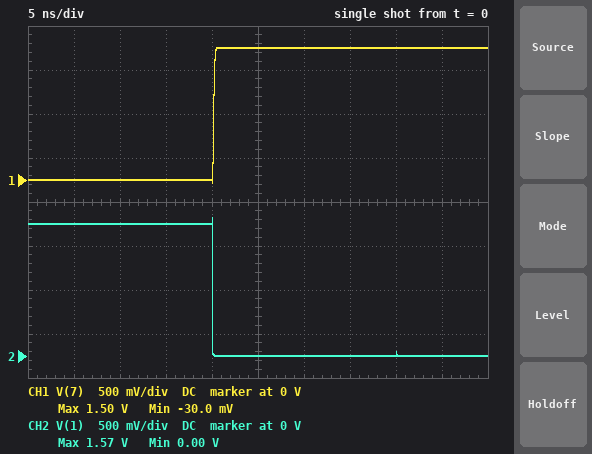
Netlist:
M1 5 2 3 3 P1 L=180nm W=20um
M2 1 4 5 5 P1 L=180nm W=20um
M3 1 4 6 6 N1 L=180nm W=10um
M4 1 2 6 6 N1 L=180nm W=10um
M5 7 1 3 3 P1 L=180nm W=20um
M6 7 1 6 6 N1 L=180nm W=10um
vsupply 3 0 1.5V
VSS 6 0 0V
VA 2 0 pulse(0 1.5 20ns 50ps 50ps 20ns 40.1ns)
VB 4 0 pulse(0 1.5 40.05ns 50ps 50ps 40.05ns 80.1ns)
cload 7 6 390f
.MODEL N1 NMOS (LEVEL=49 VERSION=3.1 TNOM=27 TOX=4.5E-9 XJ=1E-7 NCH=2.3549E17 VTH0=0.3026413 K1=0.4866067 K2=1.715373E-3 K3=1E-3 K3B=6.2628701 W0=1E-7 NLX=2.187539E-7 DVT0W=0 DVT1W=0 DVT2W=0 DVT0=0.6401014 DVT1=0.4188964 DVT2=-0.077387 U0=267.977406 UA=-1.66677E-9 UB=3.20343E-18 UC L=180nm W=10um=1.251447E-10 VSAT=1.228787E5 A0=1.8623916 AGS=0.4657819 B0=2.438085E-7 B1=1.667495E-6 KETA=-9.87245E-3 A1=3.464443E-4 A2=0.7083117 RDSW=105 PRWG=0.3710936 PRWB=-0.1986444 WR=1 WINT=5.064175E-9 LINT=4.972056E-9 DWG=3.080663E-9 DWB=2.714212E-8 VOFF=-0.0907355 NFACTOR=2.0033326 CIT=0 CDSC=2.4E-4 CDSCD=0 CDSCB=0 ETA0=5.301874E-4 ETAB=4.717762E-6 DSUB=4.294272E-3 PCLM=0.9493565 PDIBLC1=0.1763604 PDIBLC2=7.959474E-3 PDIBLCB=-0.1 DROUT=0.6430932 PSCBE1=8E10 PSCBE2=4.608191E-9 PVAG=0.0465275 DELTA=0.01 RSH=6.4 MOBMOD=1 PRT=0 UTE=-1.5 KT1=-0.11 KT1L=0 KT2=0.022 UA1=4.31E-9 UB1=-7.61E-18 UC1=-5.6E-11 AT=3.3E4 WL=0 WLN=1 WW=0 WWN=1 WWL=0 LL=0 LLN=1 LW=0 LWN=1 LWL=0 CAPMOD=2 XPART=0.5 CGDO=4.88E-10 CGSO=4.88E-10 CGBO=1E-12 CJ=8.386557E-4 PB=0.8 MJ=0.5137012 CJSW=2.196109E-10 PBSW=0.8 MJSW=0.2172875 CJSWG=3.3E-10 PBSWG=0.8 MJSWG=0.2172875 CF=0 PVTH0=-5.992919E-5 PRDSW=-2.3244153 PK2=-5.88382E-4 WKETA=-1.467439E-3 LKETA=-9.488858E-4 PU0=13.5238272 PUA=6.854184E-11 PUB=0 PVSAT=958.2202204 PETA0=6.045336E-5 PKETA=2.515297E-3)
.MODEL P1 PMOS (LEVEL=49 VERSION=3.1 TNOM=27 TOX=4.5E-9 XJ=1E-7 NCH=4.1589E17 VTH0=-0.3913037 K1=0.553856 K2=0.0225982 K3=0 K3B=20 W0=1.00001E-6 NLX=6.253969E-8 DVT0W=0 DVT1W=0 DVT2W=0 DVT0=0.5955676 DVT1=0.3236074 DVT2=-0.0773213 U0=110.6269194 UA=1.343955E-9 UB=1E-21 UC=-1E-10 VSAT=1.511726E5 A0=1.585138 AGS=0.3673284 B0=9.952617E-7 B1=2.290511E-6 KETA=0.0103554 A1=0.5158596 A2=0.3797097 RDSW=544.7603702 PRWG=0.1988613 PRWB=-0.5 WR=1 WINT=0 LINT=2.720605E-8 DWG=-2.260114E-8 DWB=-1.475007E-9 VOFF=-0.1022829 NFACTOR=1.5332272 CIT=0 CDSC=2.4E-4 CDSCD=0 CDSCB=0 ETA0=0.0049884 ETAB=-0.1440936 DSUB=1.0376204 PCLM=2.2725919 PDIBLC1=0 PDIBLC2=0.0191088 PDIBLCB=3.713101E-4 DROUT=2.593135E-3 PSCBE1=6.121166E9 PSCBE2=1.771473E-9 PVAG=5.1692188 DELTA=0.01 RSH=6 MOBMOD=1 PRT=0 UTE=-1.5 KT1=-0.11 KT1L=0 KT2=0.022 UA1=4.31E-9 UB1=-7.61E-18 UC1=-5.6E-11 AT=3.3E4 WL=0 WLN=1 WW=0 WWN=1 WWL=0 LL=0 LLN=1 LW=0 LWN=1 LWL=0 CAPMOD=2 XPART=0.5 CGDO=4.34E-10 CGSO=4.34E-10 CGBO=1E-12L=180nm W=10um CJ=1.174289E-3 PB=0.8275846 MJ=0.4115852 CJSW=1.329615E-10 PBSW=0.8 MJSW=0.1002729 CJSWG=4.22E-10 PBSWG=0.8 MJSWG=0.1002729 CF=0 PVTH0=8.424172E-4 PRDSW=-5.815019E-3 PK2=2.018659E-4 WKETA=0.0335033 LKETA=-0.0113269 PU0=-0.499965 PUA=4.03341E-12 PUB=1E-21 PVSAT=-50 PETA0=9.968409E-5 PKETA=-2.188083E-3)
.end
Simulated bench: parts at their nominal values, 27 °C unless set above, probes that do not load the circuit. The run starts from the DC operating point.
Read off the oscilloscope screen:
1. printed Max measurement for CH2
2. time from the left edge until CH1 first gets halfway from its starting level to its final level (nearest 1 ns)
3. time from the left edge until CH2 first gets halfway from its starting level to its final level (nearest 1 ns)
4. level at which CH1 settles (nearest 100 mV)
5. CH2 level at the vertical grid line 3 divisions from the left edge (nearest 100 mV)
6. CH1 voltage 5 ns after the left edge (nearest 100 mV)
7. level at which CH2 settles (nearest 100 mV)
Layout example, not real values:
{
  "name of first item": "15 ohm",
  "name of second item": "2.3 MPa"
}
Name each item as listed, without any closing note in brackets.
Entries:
{
  "printed Max measurement for CH2": "1.57 V",
  "time from the left edge until CH1 first gets halfway from its starting level to its final level": "20 ns",
  "time from the left edge until CH2 first gets halfway from its starting level to its final level": "20 ns",
  "level at which CH1 settles": "1.5 V",
  "CH2 level at the vertical grid line 3 divisions from the left edge": "1.5 V",
  "CH1 voltage 5 ns after the left edge": "0 V",
  "level at which CH2 settles": "0 V"
}
